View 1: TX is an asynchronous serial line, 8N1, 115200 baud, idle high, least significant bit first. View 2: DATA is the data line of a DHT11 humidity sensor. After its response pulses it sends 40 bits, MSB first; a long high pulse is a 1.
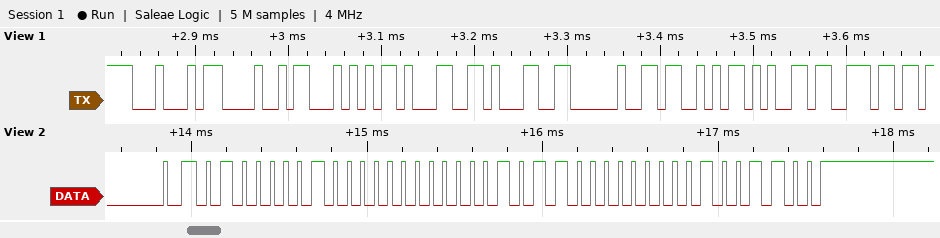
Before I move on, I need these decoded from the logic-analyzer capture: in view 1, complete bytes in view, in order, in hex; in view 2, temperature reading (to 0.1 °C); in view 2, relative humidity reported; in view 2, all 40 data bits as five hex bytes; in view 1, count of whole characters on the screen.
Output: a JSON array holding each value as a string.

["0x44 0x48 0x54 0x31 0x31 0x20 0x53 0x65 0x6E", "11.0 °C", "65 %", "41 00 0B 00 4C", "9"]
